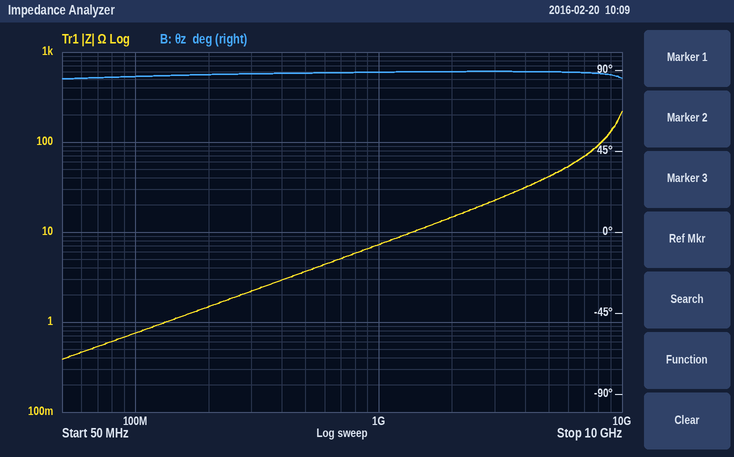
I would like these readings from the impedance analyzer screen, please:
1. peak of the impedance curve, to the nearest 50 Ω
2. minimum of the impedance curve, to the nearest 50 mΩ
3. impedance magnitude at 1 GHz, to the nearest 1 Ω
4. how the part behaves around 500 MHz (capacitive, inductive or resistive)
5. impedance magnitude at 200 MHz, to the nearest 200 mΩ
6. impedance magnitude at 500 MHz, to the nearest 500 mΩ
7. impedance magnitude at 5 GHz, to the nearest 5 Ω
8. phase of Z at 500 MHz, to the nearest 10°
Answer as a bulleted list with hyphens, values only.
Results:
- 200 Ω
- 400 mΩ
- 7 Ω
- inductive
- 1.4 Ω
- 3.5 Ω
- 40 Ω
- 90°
